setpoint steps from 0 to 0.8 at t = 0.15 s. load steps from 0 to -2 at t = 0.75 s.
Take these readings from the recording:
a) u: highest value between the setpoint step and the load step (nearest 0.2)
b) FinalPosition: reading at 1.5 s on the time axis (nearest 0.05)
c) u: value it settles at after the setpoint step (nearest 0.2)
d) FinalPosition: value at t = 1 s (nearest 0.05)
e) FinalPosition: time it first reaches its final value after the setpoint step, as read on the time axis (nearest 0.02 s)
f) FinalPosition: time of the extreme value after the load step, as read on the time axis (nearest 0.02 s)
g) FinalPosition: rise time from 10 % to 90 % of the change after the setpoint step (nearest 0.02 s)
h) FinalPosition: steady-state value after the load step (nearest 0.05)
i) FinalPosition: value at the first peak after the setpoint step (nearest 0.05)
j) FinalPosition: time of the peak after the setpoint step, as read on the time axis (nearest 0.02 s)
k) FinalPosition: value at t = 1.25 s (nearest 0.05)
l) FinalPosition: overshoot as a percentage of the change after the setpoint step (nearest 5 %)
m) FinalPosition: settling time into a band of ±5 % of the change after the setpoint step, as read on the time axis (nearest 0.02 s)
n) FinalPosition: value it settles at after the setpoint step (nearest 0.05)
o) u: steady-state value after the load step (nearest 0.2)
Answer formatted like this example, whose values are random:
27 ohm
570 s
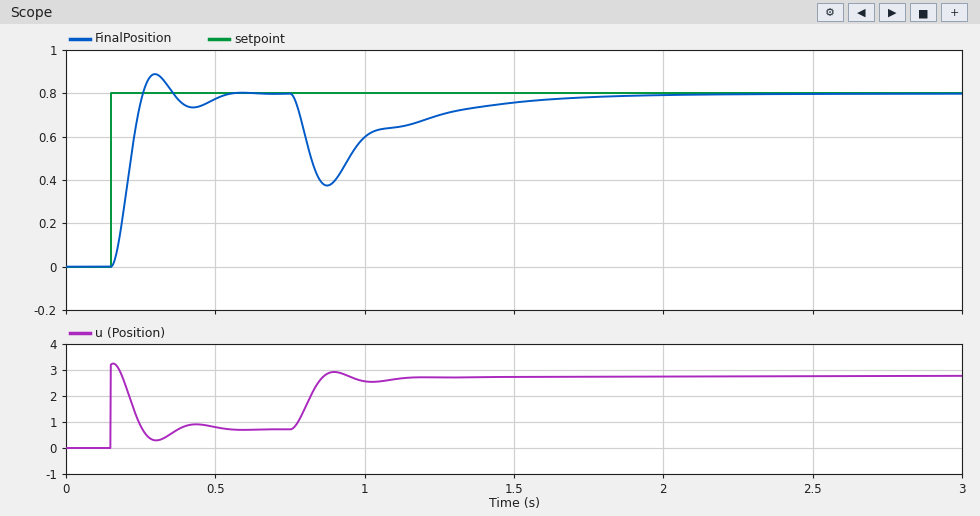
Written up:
3.2
0.75
0.8
0.60
0.26 s
0.88 s
0.08 s
0.80
0.90
0.30 s
0.70
10 %
0.48 s
0.80
2.8
